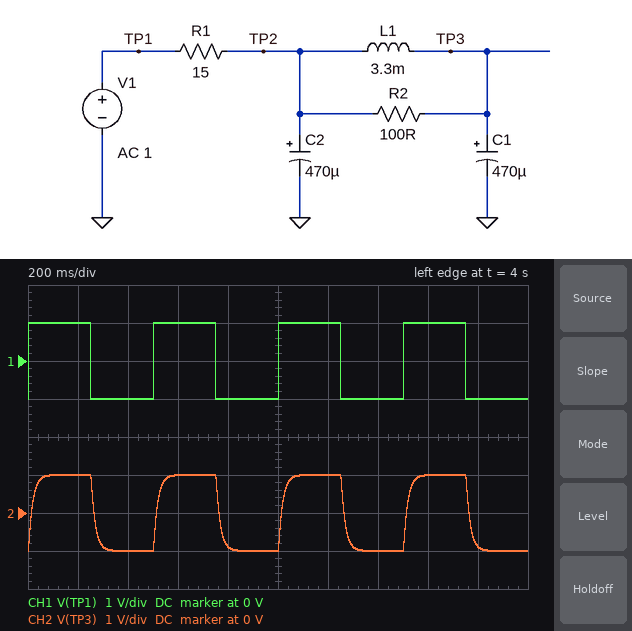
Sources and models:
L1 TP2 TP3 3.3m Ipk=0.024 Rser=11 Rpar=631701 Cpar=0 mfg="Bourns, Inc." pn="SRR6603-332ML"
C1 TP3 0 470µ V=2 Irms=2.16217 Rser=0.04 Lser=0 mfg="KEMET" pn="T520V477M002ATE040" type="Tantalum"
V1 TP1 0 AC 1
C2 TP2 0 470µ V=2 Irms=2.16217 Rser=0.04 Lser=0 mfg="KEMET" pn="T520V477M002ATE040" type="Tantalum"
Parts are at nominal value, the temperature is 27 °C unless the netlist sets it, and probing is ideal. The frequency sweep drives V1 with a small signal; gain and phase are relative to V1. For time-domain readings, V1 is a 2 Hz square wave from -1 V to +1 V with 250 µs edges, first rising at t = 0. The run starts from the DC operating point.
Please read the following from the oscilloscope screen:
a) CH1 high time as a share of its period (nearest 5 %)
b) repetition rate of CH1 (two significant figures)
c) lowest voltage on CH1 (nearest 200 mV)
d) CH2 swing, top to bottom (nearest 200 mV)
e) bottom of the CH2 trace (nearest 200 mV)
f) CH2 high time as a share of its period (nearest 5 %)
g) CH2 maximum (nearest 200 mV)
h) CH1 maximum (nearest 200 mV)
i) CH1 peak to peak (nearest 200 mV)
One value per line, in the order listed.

50 %
2.0 Hz
-1.0 V
2.0 V
-1.0 V
50 %
1.0 V
1.0 V
2.0 V
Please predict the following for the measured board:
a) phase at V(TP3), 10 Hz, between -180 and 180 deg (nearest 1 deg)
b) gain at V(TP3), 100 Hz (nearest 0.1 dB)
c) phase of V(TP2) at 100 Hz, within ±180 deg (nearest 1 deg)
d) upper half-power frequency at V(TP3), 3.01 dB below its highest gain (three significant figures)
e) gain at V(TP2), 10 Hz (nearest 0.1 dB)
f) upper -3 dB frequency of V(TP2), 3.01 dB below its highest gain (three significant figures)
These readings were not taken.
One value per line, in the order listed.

-54 deg
-24.0 dB
-62 deg
9.39 Hz
-3.0 dB
10.1 Hz
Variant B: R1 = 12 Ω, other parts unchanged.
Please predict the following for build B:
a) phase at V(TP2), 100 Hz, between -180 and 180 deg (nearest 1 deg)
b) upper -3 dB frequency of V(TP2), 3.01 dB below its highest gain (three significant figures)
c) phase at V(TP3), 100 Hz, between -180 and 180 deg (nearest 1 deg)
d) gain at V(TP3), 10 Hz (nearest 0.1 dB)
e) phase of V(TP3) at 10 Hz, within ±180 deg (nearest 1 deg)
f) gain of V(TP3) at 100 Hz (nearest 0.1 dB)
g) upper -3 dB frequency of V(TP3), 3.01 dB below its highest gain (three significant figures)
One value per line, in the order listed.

-59 deg
12.4 Hz
-139 deg
-2.5 dB
-48 deg
-22.3 dB
11.2 Hz
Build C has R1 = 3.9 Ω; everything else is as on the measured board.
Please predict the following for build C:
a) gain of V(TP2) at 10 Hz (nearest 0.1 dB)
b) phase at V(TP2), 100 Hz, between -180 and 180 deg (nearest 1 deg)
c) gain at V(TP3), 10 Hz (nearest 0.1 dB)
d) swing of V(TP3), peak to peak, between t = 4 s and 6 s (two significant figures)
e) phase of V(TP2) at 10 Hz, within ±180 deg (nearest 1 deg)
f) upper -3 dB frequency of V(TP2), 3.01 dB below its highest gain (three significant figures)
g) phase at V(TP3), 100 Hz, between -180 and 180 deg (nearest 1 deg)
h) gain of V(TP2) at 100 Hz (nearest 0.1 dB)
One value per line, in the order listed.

-0.5 dB
-41 deg
-0.8 dB
2.0 V
-12 deg
41.0 Hz
-121 deg
-5.3 dB
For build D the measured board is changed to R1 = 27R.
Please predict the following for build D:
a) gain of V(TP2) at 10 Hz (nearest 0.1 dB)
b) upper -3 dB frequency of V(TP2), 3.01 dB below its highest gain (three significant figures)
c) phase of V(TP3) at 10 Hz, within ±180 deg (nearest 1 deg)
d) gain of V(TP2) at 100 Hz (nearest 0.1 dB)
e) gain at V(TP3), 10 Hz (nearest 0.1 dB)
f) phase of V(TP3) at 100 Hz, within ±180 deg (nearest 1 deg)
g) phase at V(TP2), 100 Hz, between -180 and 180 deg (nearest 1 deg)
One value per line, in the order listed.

-5.8 dB
5.82 Hz
-68 deg
-19.3 dB
-6.2 dB
-146 deg
-66 deg
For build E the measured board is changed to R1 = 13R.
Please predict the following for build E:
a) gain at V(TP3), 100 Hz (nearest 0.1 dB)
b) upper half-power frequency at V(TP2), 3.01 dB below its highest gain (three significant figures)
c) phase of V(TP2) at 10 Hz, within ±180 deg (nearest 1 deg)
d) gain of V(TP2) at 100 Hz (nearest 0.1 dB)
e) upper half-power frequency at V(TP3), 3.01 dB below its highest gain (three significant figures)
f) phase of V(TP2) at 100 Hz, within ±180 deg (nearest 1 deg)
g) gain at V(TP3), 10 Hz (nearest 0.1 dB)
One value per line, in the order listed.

-22.9 dB
11.5 Hz
-34 deg
-13.4 dB
10.5 Hz
-60 deg
-2.8 dB
